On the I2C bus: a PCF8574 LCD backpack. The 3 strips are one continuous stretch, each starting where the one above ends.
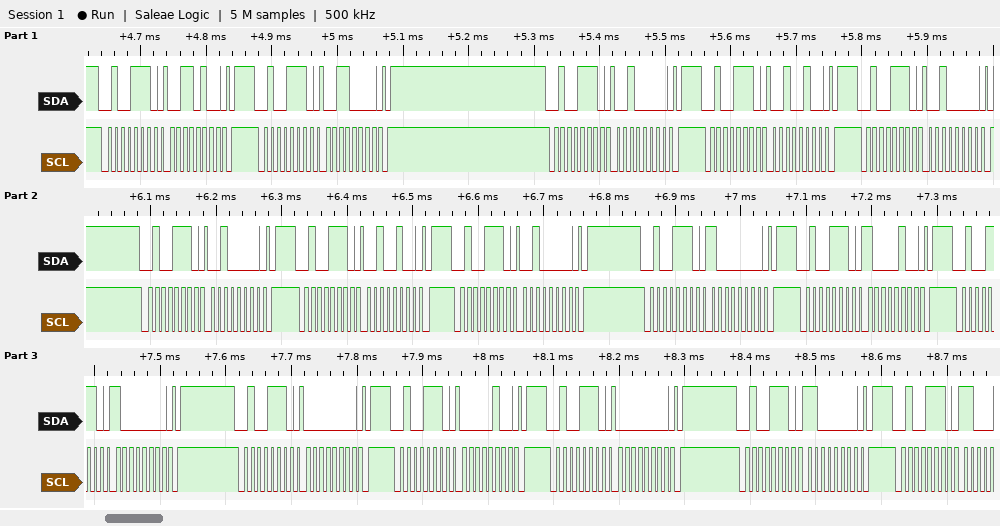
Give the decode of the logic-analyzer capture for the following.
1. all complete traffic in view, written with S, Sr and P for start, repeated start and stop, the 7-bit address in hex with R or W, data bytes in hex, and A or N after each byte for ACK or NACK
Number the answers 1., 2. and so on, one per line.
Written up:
1. S 27W A 34 A P S 27W A 30 A P S 27W A 20 A P S 27W A 24 A P S 27W A 20 A P S 27W A 20 A P S 27W A 24 A P S 27W A 20 A P S 27W A 80 A P S 27W A 84 A P S 27W A 80 A P S 27W A 00 A P S 27W A 04 A P S 27W A 00 A P S 27W A C0 A P S 27W A
